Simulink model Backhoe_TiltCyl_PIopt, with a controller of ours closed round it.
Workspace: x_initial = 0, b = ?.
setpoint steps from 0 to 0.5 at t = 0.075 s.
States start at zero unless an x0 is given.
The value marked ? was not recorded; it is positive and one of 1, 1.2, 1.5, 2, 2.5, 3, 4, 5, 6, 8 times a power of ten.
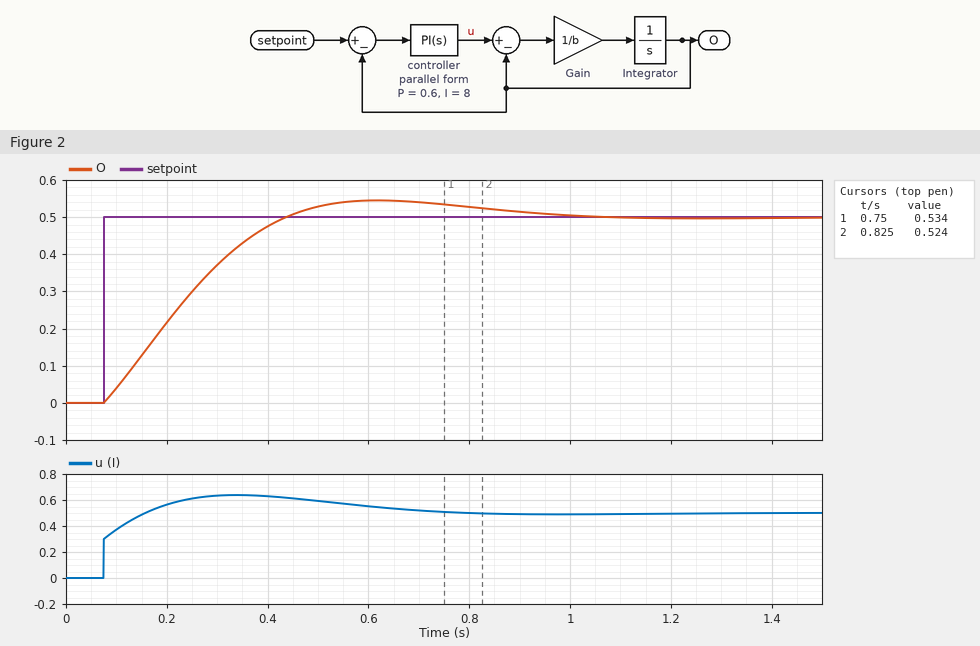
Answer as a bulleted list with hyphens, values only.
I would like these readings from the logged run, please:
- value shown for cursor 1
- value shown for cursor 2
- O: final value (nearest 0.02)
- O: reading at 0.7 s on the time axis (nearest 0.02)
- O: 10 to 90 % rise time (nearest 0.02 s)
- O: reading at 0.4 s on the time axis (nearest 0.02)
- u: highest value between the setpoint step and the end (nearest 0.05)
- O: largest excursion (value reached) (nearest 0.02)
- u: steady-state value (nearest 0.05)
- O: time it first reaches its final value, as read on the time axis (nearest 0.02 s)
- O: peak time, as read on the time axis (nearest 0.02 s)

- 0.534
- 0.524
- 0.50
- 0.54
- 0.26 s
- 0.48
- 0.65
- 0.54
- 0.50
- 0.44 s
- 0.62 s
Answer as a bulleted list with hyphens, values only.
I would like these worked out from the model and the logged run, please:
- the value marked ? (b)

- 0.2
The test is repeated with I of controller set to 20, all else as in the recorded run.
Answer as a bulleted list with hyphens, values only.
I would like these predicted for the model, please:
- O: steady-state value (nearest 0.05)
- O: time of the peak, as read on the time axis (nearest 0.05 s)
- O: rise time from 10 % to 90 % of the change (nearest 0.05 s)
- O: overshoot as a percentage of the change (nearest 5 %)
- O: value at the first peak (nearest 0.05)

- 0.50
- 0.40 s
- 0.15 s
- 25 %
- 0.65
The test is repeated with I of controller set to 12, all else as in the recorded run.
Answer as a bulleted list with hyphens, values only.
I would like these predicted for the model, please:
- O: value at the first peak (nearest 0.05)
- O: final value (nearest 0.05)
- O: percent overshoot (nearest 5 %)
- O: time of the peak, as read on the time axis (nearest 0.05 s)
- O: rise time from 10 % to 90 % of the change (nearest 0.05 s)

- 0.60
- 0.50
- 15 %
- 0.50 s
- 0.20 s
